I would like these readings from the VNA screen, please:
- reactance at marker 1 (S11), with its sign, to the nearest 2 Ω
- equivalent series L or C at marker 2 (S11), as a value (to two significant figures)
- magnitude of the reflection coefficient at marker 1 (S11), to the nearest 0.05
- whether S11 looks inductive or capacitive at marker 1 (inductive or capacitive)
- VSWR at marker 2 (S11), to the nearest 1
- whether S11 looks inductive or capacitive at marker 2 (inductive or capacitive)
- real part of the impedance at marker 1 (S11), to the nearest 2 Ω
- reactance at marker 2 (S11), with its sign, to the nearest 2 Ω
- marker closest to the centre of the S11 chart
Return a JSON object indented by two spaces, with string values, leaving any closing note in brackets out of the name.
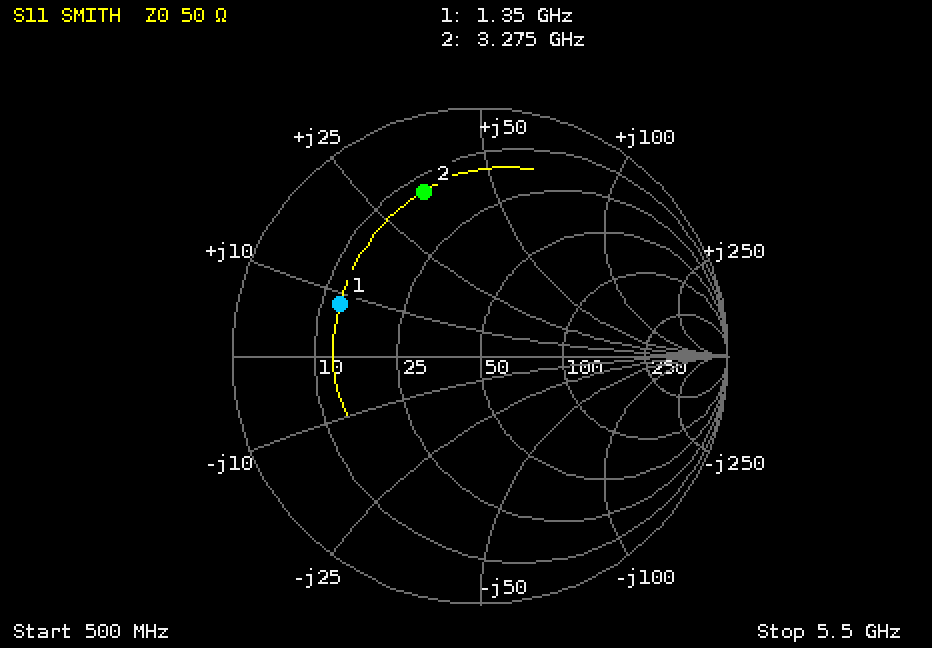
{
  "reactance at marker 1 (S11), with its sign, to the nearest 2 Ω": "+8 Ω",
  "equivalent series L or C at marker 2 (S11), as a value": "1.7 nH",
  "magnitude of the reflection coefficient at marker 1 (S11), to the nearest 0.05": "0.60",
  "whether S11 looks inductive or capacitive at marker 1": "inductive",
  "VSWR at marker 2 (S11), to the nearest 1": "6",
  "whether S11 looks inductive or capacitive at marker 2": "inductive",
  "real part of the impedance at marker 1 (S11), to the nearest 2 Ω": "12 Ω",
  "reactance at marker 2 (S11), with its sign, to the nearest 2 Ω": "+34 Ω",
  "marker closest to the centre of the S11 chart": "marker 1"
}
